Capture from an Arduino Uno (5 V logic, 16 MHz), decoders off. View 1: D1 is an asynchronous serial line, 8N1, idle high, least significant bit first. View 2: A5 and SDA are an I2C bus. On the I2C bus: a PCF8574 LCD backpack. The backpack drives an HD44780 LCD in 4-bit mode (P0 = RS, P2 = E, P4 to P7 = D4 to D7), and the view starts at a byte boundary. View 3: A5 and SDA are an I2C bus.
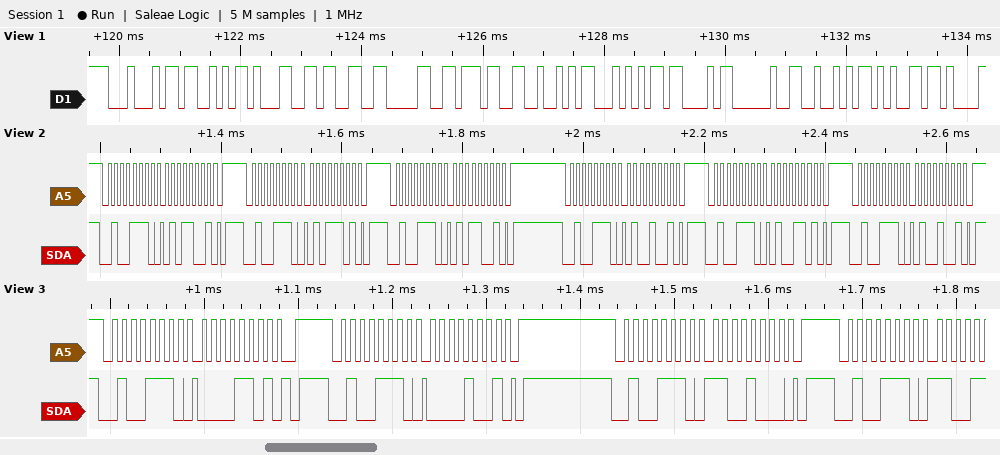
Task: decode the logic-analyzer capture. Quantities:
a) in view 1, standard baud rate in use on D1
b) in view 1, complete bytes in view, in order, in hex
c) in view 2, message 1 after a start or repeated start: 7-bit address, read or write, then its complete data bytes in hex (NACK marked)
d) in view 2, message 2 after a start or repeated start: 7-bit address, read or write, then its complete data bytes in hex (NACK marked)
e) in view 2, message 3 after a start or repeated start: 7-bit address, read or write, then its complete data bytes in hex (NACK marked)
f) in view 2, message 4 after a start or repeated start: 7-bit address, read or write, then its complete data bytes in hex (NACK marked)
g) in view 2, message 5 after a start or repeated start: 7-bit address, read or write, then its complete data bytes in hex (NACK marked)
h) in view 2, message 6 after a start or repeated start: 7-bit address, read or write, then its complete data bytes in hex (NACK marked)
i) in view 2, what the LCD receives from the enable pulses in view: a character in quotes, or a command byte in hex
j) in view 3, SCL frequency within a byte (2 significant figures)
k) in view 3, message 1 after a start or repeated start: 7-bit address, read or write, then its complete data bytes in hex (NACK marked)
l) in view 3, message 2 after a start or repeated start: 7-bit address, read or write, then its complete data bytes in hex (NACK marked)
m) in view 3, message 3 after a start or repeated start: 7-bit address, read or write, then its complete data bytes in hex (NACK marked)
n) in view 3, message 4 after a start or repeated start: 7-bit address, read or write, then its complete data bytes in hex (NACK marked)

9600 baud
44 53 31 33 30 37 52 54 43 20 52 65
0x27 write: 59
0x27 write: 5D
0x27 write: 59
0x27 write: 49
0x27 write: 4D
0x27 write: 49
'T'
100 kHz
0x27 write: 0D
0x27 write: 09
0x27 write: C8
0x27 write
